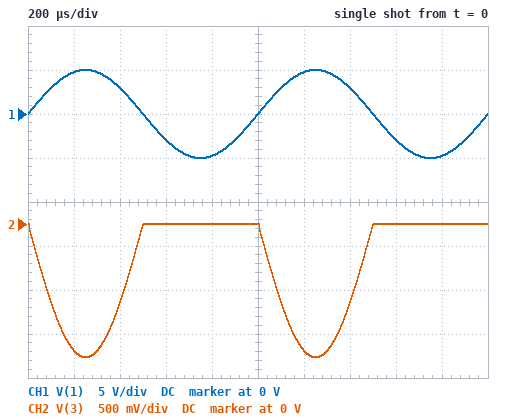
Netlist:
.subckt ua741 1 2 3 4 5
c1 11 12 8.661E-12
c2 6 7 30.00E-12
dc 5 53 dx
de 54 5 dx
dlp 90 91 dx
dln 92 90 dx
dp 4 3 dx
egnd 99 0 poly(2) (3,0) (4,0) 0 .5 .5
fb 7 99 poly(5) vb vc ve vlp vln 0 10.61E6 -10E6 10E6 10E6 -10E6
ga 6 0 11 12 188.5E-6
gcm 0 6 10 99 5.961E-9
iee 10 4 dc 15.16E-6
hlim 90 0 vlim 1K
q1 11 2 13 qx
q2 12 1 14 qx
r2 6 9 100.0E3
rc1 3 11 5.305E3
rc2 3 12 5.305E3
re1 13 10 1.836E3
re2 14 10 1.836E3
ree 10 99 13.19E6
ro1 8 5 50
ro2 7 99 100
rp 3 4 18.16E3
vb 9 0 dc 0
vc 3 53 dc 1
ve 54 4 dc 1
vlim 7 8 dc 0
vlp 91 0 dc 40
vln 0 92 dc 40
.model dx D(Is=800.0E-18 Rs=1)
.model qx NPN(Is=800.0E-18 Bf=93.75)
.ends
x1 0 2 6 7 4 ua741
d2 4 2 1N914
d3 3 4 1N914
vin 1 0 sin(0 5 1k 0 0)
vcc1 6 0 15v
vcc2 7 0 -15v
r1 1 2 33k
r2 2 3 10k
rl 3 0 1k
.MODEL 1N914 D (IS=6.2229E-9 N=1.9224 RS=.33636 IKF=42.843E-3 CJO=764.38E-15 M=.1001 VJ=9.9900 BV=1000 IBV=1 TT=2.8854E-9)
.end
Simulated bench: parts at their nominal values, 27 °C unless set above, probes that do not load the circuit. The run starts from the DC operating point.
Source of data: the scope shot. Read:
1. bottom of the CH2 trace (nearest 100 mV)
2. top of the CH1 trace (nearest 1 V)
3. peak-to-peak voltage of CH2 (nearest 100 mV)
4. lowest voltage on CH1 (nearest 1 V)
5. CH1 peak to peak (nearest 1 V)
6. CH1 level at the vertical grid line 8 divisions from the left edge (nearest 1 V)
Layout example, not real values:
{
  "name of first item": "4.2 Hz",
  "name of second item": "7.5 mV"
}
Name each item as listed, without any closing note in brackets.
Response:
{
  "bottom of the CH2 trace": "-1.5 V",
  "top of the CH1 trace": "5 V",
  "peak-to-peak voltage of CH2": "1.5 V",
  "lowest voltage on CH1": "-5 V",
  "CH1 peak to peak": "10 V",
  "CH1 level at the vertical grid line 8 divisions from the left edge": "-3 V"
}
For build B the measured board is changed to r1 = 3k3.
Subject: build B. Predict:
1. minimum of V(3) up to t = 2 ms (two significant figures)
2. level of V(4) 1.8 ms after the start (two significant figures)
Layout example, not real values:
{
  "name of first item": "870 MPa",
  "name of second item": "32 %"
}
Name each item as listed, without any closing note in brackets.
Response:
{
  "minimum of V(3) up to t = 2 ms": "-14 V",
  "level of V(4) 1.8 ms after the start": "620 mV"
}
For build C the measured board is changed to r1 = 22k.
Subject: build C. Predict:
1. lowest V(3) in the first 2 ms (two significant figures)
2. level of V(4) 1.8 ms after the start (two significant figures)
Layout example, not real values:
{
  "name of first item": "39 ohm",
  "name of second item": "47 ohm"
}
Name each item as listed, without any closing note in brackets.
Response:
{
  "lowest V(3) in the first 2 ms": "-2.3 V",
  "level of V(4) 1.8 ms after the start": "520 mV"
}
